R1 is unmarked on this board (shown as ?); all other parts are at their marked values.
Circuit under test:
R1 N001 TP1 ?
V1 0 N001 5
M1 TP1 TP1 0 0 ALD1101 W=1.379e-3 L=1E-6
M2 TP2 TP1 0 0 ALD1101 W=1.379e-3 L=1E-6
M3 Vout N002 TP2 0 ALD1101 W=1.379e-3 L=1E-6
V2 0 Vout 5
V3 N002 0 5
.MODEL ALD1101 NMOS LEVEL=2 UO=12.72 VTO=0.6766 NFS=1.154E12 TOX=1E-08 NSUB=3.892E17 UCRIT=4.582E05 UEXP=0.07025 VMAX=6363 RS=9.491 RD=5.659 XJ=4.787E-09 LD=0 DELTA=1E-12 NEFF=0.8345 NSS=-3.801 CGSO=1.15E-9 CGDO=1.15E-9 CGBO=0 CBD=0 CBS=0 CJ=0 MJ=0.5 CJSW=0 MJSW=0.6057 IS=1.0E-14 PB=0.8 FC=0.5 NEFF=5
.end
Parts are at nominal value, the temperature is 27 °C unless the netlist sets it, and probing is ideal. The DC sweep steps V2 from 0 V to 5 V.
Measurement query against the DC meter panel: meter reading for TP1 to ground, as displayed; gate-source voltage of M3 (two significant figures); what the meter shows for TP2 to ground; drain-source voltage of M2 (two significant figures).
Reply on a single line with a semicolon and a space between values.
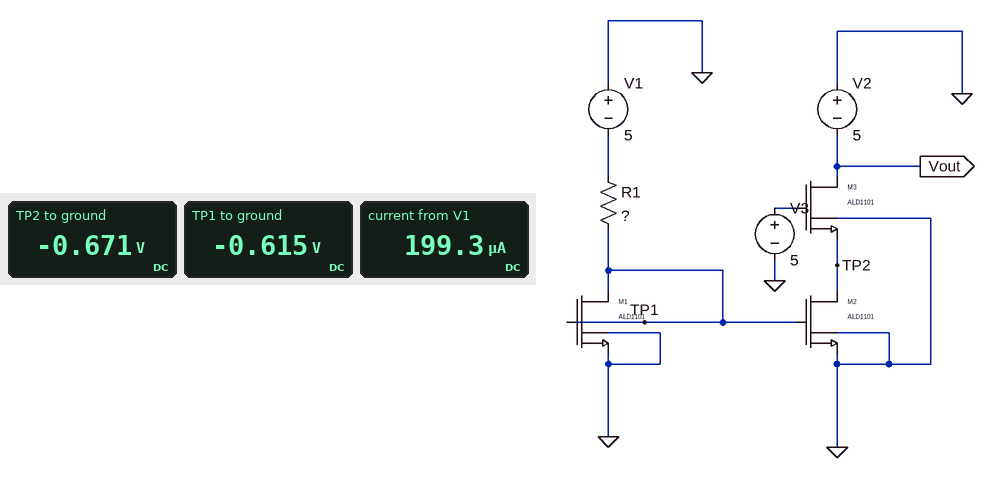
-0.615 V; 5.7 V; -0.671 V; -670 mV
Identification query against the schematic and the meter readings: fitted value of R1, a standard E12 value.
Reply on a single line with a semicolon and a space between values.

22 kΩ
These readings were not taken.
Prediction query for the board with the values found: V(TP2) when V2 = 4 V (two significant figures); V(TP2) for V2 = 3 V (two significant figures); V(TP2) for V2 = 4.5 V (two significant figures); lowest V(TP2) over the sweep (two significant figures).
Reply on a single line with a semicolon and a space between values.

-670 mV; -670 mV; -670 mV; -670 mV
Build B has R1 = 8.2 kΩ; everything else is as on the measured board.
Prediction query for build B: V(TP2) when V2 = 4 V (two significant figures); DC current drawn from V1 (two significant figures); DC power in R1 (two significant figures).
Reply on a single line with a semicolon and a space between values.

-670 mV; 530 µA; 2.3 mW
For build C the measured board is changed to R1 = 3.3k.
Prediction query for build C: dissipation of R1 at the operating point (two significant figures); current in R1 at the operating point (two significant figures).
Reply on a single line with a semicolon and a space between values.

5.7 mW; 1.3 mA
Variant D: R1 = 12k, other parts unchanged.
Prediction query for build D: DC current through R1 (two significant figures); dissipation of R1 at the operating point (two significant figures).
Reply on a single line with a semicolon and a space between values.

360 µA; 1.6 mW
